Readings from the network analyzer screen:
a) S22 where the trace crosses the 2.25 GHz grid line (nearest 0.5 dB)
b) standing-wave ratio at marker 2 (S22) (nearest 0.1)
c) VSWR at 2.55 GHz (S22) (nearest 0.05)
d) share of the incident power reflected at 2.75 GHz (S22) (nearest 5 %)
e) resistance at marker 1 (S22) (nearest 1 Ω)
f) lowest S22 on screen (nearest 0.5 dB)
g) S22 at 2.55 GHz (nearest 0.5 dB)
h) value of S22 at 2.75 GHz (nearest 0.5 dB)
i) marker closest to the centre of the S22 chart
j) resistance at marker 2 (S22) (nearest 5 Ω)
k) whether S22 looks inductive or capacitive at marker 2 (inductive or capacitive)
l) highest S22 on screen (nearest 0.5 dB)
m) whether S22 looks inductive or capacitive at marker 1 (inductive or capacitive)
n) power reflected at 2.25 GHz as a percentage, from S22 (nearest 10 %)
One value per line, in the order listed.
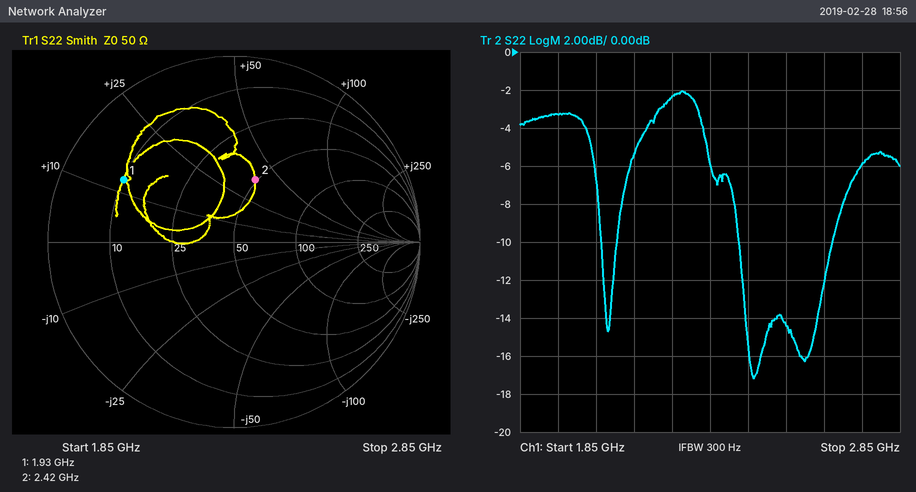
-2.5 dB
2.1
1.45
25 %
10 Ω
-17.0 dB
-14.5 dB
-6.0 dB
marker 2
50 Ω
inductive
-2.0 dB
inductive
60 %
